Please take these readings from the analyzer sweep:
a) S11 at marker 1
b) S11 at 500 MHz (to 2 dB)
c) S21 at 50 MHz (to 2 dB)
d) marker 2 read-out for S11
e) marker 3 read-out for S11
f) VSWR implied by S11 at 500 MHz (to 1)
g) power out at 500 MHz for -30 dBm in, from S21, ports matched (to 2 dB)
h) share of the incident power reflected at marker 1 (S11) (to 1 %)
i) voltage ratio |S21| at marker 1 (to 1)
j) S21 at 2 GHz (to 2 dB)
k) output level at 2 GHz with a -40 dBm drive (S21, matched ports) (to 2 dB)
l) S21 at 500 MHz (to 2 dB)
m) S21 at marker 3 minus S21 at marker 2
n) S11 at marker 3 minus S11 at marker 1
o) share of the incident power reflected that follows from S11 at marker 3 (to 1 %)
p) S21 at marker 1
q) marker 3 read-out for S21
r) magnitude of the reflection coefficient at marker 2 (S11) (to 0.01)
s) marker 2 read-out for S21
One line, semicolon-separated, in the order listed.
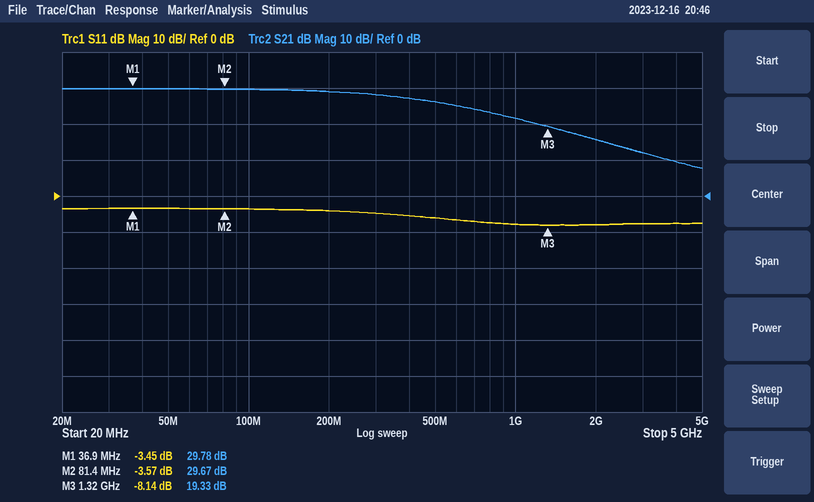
-3.45 dB; -6 dB; 30 dB; -3.57 dB; -8.14 dB; 3; -4 dBm; 45 %; 31; 16 dB; -24 dBm; 26 dB; -10.34 dB; -4.69 dB; 15 %; 29.78 dB; 19.33 dB; 0.66; 29.67 dB
